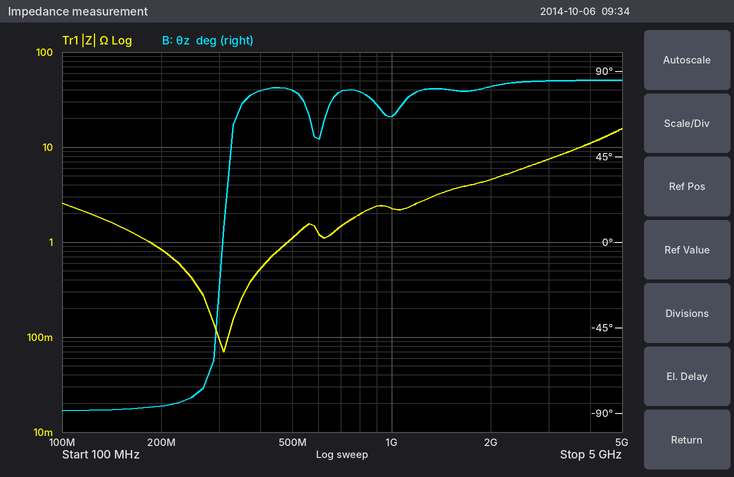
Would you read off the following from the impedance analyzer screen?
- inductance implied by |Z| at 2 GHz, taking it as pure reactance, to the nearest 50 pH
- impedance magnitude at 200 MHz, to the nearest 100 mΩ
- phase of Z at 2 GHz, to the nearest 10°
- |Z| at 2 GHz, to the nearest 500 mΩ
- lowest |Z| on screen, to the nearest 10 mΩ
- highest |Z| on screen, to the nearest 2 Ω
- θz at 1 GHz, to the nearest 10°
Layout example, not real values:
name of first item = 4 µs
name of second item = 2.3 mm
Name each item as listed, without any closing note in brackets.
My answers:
inductance implied by |Z| at 2 GHz, taking it as pure reactance, to the nearest 50 pH = 350 pH
impedance magnitude at 200 MHz, to the nearest 100 mΩ = 800 mΩ
phase of Z at 2 GHz, to the nearest 10° = 80°
|Z| at 2 GHz, to the nearest 500 mΩ = 4.5 Ω
lowest |Z| on screen, to the nearest 10 mΩ = 70 mΩ
highest |Z| on screen, to the nearest 2 Ω = 16 Ω
θz at 1 GHz, to the nearest 10° = 70°
